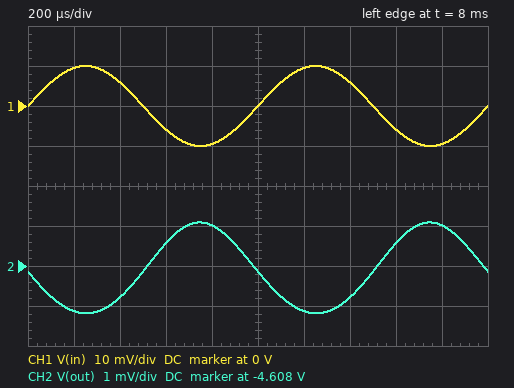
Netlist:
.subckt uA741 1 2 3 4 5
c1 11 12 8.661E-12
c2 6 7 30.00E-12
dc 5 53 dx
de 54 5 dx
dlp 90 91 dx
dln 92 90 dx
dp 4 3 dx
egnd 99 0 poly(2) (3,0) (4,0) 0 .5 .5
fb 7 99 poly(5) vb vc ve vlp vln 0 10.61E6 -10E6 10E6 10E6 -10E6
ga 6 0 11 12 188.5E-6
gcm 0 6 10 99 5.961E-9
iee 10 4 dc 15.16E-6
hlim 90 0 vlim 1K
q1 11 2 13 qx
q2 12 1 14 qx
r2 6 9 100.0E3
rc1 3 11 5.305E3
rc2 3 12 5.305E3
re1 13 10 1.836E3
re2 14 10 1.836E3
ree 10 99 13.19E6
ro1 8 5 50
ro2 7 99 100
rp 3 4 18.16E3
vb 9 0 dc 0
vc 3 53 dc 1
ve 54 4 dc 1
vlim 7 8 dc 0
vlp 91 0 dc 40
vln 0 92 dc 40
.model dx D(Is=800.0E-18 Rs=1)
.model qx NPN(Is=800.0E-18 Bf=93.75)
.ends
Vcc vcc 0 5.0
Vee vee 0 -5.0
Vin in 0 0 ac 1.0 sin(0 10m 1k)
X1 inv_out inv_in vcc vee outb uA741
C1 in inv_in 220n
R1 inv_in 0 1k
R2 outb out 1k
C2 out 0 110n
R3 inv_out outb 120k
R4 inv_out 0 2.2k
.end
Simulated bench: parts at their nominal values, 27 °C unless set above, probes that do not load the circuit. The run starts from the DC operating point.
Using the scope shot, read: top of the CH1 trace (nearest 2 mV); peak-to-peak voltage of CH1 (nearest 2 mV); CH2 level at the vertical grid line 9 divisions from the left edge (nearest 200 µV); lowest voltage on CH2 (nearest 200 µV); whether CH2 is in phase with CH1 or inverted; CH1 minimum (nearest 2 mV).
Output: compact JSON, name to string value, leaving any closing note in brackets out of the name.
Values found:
{"top of the CH1 trace": "10 mV", "peak-to-peak voltage of CH1": "20 mV", "CH2 level at the vertical grid line 9 divisions from the left edge": "-4.6070 V", "lowest voltage on CH2": "-4.6092 V", "whether CH2 is in phase with CH1 or inverted": "inverted", "CH1 minimum": "-10 mV"}
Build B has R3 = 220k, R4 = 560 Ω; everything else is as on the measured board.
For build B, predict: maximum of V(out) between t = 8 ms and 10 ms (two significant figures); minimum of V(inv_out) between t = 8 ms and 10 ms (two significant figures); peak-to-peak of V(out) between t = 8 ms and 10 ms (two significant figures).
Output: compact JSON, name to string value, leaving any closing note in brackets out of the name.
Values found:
{"maximum of V(out) between t = 8 ms and 10 ms": "-4.5 V", "minimum of V(inv_out) between t = 8 ms and 10 ms": "-12 mV", "peak-to-peak of V(out) between t = 8 ms and 10 ms": "36 mV"}
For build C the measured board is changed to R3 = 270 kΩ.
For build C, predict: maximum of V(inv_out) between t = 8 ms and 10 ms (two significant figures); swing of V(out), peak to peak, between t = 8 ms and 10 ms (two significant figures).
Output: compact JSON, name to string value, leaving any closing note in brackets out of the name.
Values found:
{"maximum of V(inv_out) between t = 8 ms and 10 ms": "-37 mV", "swing of V(out), peak to peak, between t = 8 ms and 10 ms": "8.6 mV"}
